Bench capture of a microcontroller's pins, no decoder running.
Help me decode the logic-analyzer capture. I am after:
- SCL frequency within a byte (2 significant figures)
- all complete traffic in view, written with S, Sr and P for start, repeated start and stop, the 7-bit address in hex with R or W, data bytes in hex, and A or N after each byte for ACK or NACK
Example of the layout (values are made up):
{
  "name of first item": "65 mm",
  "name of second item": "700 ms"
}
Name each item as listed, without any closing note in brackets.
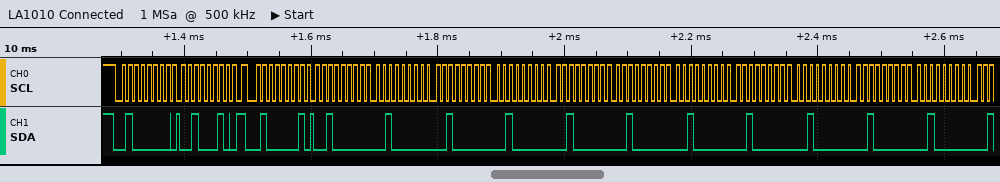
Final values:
{
  "SCL frequency within a byte": "100 kHz",
  "all complete traffic in view, written with S, Sr and P for start, repeated start and stop, the 7-bit address in hex with R or W, data bytes in hex, and A or N after each byte for ACK or NACK": "S 20W A 22 A Sr 20R A 20 A 20 A 20 A 20 A 20 A 20 A 20 A 20 A 20 A 20 A 20 A"
}
